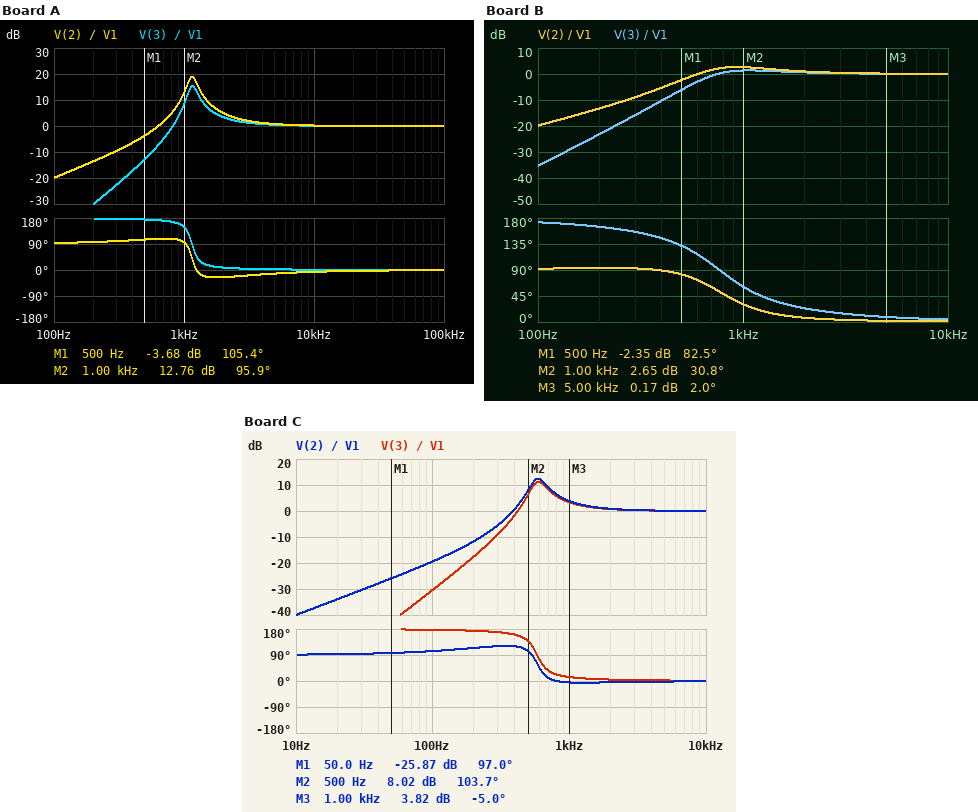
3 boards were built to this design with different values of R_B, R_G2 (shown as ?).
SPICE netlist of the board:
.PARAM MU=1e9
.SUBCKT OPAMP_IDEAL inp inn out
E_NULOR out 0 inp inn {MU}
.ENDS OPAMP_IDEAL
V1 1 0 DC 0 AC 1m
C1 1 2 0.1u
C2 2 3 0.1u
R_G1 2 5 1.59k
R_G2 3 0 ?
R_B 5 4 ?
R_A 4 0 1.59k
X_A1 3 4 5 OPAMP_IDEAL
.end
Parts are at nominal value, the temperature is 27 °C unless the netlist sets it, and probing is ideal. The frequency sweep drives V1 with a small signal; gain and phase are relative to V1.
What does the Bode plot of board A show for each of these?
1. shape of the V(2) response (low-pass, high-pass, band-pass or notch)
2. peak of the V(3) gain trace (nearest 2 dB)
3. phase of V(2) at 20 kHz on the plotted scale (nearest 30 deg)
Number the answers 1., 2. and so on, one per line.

1. high-pass
2. 16 dB
3. 0 deg
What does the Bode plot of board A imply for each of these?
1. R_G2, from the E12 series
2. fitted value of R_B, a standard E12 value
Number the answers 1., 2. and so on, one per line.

1. 1.2 kΩ
2. 3.9 kΩ
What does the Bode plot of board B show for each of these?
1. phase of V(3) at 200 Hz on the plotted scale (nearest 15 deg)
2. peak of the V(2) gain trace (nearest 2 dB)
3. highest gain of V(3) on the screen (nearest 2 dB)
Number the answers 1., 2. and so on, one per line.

1. 165 deg
2. 2 dB
3. 2 dB
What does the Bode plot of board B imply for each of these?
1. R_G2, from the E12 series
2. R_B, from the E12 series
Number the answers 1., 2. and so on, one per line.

1. 2.7 kΩ
2. 680 Ω
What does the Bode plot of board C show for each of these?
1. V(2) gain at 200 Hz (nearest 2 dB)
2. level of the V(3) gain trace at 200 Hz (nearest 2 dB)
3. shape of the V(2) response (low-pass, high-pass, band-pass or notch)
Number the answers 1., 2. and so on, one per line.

1. -12 dB
2. -18 dB
3. high-pass
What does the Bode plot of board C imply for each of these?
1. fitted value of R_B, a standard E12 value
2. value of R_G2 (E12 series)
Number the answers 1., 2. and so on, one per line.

1. 820 Ω
2. 4.7 kΩ
